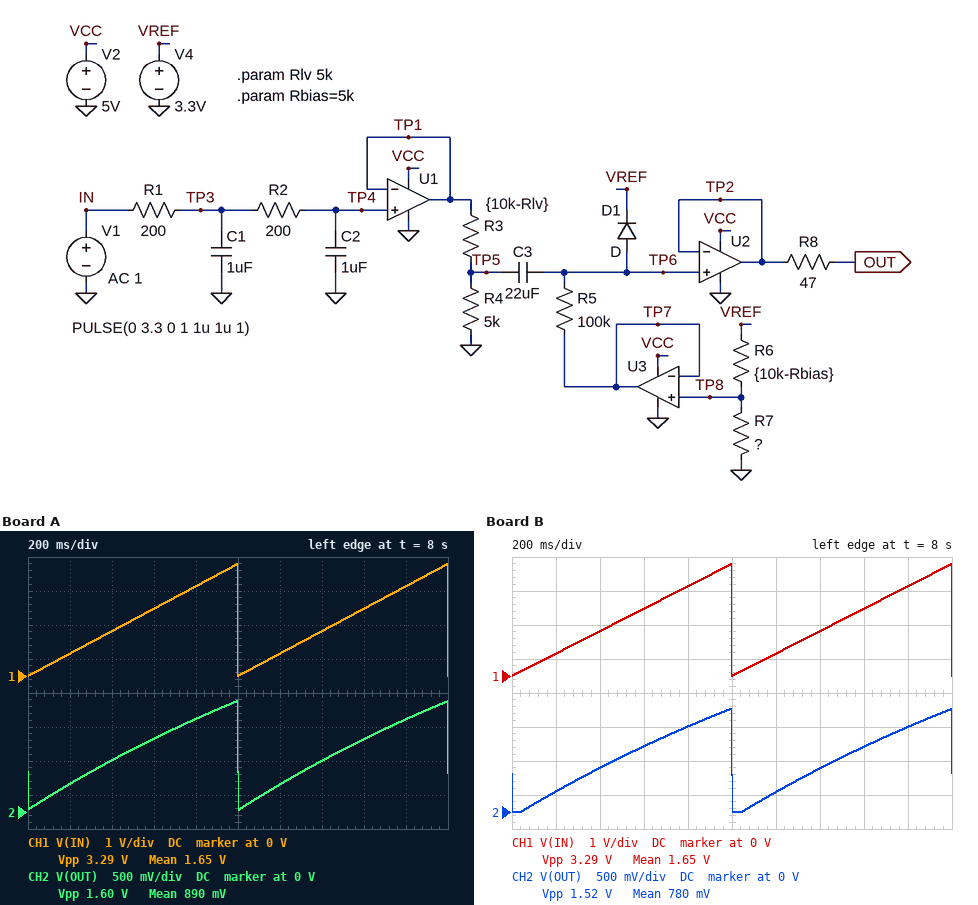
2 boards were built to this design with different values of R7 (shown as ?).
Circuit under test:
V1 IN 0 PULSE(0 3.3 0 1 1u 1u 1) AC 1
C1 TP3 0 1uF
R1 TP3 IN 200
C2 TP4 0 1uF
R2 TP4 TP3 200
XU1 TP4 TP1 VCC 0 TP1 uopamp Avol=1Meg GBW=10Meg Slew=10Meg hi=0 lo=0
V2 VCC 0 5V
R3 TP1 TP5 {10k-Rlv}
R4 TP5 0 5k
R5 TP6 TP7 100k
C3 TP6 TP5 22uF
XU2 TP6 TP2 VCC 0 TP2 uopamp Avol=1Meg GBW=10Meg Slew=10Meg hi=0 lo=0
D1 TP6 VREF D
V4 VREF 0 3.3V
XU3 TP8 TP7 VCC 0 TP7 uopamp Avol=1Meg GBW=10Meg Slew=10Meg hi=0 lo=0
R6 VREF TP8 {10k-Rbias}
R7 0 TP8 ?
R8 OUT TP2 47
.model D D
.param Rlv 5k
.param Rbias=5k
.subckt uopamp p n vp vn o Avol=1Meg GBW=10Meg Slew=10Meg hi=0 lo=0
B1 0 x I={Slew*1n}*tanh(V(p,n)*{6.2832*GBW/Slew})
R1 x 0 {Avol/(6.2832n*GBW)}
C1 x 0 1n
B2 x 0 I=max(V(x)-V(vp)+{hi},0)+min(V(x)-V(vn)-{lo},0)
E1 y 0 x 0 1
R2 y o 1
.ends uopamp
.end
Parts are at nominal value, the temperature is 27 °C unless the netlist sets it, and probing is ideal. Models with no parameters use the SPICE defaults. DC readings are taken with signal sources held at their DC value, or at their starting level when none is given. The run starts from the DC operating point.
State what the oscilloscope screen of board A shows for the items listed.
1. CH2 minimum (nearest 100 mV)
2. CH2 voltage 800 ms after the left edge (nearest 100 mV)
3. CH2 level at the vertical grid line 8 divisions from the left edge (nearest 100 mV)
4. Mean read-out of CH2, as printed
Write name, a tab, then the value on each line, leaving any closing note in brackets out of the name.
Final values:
CH2 minimum	0 V
CH2 voltage 800 ms after the left edge	1.4 V
CH2 level at the vertical grid line 8 divisions from the left edge	1.1 V
Mean read-out of CH2, as printed	890 mV
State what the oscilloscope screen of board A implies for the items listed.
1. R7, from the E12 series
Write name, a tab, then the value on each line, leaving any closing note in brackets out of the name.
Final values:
R7, from the E12 series	1.8 kΩ
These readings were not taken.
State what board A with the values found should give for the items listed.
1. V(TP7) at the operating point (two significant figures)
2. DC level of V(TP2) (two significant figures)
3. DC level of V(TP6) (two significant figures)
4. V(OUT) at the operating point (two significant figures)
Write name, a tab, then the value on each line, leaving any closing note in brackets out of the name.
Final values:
V(TP7) at the operating point	870 mV
DC level of V(TP2)	870 mV
DC level of V(TP6)	870 mV
V(OUT) at the operating point	870 mV
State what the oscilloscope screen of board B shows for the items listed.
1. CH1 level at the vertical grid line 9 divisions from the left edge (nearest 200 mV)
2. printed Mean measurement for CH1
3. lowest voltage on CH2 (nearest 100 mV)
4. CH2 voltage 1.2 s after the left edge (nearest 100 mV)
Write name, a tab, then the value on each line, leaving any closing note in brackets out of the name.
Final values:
CH1 level at the vertical grid line 9 divisions from the left edge	2.6 V
printed Mean measurement for CH1	1.65 V
lowest voltage on CH2	0 V
CH2 voltage 1.2 s after the left edge	300 mV
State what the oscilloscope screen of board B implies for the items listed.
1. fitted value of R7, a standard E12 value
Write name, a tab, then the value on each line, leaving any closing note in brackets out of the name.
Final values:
fitted value of R7, a standard E12 value	1.5 kΩ
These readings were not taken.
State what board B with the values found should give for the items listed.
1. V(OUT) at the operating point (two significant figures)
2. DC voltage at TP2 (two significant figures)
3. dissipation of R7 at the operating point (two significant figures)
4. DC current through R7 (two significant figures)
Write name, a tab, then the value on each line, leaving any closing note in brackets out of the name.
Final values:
V(OUT) at the operating point	760 mV
DC voltage at TP2	760 mV
dissipation of R7 at the operating point	390 µW
DC current through R7	510 µA
